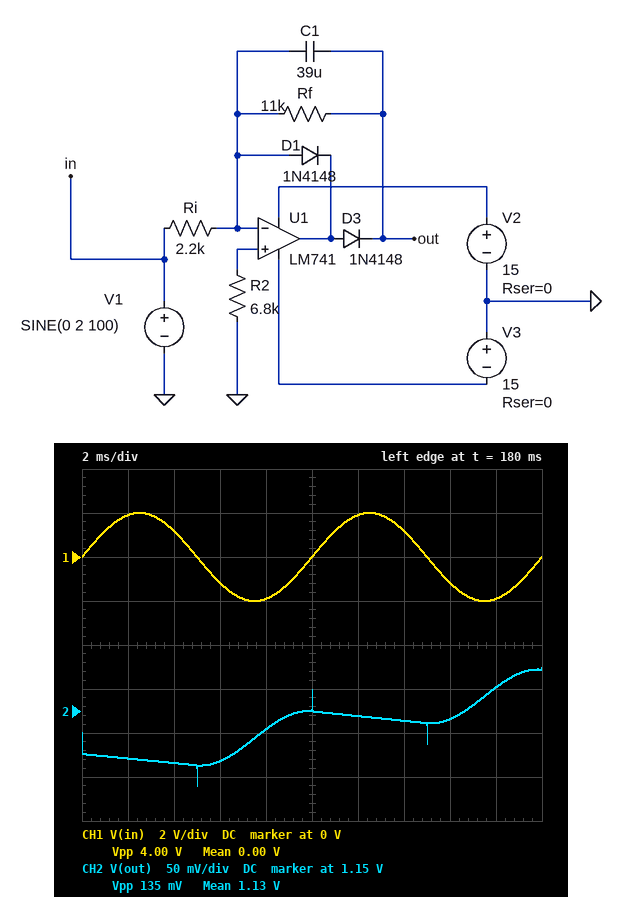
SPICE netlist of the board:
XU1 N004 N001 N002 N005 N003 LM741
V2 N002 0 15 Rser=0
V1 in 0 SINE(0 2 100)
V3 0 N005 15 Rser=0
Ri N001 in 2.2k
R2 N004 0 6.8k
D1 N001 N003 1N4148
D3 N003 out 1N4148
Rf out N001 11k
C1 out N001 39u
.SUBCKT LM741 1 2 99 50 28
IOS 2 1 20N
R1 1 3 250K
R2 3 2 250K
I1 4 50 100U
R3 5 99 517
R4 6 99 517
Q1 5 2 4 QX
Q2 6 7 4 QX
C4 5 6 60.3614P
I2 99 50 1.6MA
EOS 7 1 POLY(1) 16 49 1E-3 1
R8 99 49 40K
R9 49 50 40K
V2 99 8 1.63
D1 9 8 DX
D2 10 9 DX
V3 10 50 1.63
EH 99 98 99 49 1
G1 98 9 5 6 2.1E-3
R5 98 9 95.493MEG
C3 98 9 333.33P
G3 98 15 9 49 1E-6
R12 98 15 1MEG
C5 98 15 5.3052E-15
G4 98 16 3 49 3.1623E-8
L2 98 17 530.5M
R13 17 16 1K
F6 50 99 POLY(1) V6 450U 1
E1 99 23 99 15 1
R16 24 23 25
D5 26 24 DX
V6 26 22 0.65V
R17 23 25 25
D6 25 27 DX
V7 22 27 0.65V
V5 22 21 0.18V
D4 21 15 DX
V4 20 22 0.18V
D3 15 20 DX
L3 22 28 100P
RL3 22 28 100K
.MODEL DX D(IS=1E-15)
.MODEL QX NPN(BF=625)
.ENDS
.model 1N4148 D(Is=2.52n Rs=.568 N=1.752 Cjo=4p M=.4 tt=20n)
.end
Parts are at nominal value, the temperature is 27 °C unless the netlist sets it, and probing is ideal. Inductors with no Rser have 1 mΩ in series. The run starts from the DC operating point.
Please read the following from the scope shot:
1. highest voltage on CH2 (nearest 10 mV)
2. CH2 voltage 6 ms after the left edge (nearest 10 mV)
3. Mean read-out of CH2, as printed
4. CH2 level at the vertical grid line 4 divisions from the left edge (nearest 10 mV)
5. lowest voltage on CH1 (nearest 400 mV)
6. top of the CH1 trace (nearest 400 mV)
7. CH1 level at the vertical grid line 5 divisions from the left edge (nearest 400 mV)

1.20 V
1.09 V
1.13 V
1.13 V
-2.0 V
2.0 V
0 V
